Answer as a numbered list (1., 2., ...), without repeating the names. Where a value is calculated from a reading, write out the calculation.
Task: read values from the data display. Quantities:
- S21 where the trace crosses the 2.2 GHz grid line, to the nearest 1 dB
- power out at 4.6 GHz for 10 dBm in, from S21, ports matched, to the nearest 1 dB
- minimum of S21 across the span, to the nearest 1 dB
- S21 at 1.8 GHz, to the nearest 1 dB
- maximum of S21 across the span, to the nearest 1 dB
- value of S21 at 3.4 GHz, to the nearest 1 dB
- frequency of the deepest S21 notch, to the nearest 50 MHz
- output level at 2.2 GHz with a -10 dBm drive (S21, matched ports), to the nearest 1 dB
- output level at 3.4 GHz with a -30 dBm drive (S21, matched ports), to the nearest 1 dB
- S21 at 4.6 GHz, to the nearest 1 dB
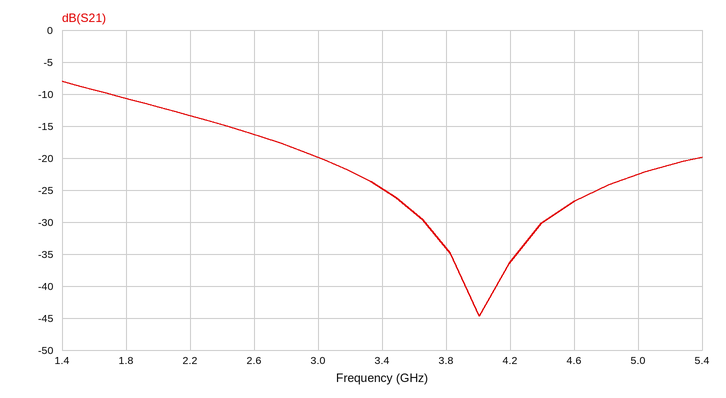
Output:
1. -13 dB
2. 10 dBm + (-27 dB) = -17 dBm
3. -45 dB
4. -11 dB
5. -8 dB
6. -25 dB
7. 4.00 GHz
8. -10 dBm + (-13 dB) = -23 dBm
9. -30 dBm + (-25 dB) = -55 dBm
10. -27 dB
